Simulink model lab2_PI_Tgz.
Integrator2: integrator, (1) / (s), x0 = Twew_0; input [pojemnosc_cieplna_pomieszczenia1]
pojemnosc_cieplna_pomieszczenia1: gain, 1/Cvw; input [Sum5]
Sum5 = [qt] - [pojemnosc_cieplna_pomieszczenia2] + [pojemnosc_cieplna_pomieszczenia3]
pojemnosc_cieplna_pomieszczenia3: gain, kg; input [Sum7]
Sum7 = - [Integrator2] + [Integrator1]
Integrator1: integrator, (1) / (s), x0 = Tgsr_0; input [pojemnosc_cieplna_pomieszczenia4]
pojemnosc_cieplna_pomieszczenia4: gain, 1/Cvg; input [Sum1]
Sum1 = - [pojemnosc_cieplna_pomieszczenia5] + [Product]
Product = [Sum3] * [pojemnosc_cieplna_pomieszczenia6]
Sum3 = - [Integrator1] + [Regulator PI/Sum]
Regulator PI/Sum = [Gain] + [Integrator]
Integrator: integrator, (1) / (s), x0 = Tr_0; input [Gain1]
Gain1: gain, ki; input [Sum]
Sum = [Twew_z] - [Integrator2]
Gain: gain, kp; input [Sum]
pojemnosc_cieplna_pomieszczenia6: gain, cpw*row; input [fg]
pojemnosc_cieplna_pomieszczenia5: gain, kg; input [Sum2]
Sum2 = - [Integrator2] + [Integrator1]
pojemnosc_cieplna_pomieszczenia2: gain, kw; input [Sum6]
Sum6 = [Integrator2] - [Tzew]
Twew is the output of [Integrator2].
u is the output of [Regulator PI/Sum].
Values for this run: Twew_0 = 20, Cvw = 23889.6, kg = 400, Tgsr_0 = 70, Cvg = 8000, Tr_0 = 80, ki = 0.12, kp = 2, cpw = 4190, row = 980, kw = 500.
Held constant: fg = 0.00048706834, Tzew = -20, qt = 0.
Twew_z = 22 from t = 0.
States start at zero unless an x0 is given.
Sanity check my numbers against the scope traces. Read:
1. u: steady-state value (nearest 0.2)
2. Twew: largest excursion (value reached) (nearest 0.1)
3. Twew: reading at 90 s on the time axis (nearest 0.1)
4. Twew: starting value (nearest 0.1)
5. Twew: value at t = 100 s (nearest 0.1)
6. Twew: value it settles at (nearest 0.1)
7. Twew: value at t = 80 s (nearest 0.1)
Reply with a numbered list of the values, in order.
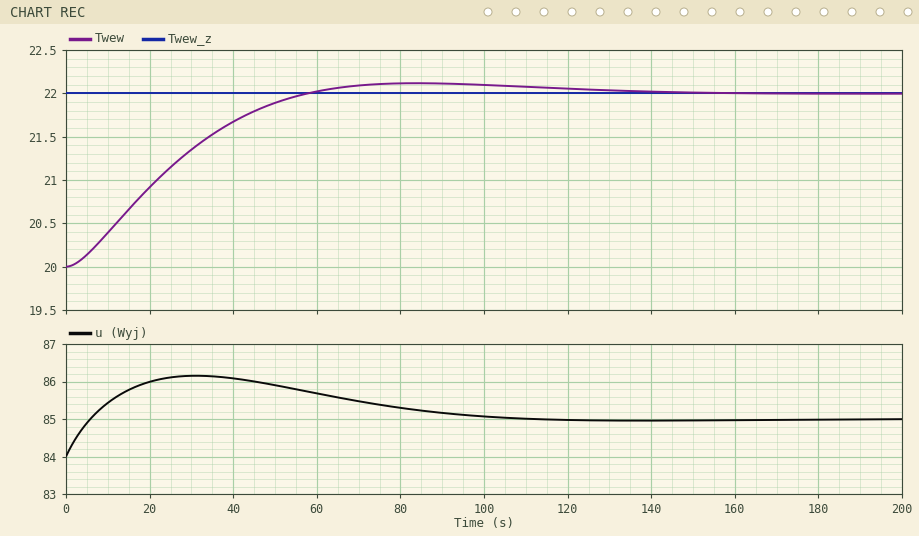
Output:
1. 85.0
2. 22.1
3. 22.1
4. 20.0
5. 22.1
6. 22.0
7. 22.1
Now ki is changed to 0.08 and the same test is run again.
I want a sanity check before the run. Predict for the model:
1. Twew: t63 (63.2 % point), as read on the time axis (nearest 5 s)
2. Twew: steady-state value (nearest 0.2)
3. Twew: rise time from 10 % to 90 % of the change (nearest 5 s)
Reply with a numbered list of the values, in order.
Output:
1. 35 s
2. 22.0
3. 60 s
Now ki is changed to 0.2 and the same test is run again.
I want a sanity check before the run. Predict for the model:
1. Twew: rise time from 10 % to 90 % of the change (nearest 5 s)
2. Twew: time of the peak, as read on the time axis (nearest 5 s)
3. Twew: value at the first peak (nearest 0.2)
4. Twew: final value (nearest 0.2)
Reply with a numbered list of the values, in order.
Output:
1. 25 s
2. 60 s
3. 22.4
4. 22.0
